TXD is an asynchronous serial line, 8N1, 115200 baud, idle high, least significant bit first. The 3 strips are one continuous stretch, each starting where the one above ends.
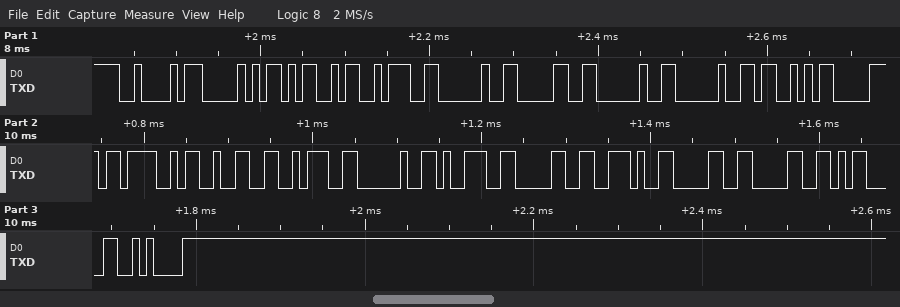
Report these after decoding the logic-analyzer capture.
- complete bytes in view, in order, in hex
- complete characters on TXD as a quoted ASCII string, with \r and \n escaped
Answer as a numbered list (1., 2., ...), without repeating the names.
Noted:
1. 0x42 0x50 0x4D 0x3A 0x20 0x30 0x20 0x20 0x53 0x70 0x4F 0x32 0x3A 0x20 0x39 0x30 0x2E 0x30 0x30 0x0D 0x0A
2. "BPM: 0  SpO2: 90.00\r\n"
